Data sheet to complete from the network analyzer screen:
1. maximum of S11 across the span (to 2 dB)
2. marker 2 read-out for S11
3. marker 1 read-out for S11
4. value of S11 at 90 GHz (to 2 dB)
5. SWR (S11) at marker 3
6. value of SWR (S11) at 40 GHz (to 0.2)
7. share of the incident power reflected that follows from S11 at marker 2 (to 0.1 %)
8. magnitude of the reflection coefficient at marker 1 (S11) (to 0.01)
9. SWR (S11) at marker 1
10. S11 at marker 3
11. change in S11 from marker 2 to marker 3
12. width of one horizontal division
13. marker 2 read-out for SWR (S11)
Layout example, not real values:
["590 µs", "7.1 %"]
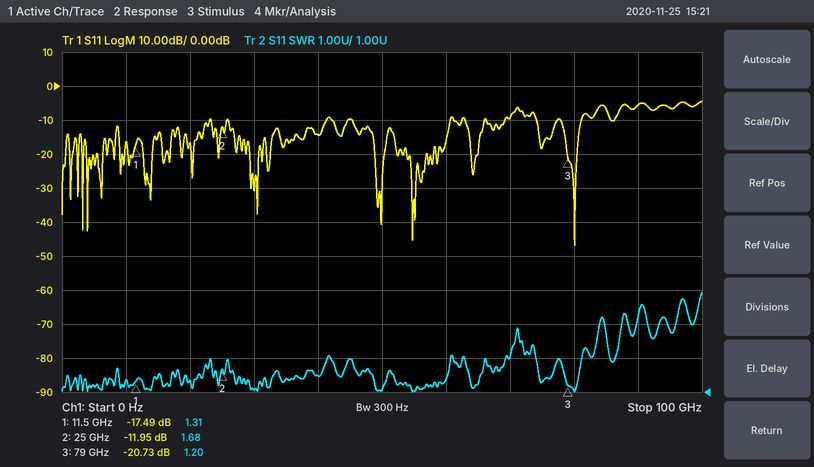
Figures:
["-4 dB", "-11.95 dB", "-17.49 dB", "-6 dB", "1.20", "1.4", "6.4 %", "0.13", "1.31", "-20.73 dB", "-8.78 dB", "10 GHz", "1.68"]
